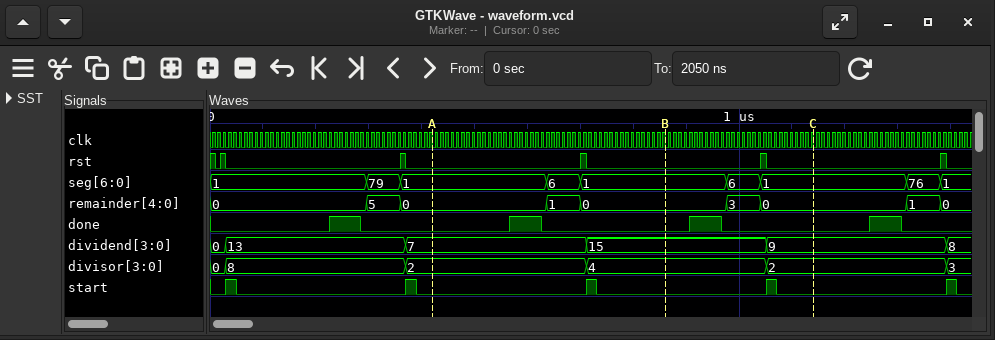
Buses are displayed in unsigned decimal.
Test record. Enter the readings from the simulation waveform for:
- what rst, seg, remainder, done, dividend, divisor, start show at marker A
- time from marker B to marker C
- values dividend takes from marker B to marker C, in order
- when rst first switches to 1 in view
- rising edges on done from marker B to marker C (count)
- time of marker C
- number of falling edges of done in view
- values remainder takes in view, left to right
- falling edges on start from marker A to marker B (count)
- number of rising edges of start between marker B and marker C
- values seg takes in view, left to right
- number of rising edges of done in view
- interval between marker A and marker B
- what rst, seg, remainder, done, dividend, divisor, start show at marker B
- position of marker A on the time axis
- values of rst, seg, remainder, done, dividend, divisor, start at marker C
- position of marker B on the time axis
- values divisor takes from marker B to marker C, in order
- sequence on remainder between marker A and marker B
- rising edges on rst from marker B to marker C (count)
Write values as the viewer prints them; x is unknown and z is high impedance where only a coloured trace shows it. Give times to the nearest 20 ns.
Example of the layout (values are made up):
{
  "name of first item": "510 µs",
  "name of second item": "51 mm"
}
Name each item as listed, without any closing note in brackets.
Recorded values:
{
  "what rst, seg, remainder, done, dividend, divisor, start show at marker A": "rst=0, seg=1, remainder=0, done=0, dividend=7, divisor=2, start=0",
  "time from marker B to marker C": "280 ns",
  "values dividend takes from marker B to marker C, in order": "15, 9",
  "when rst first switches to 1 in view": "20 ns",
  "rising edges on done from marker B to marker C": "1",
  "time of marker C": "1140 ns",
  "number of falling edges of done in view": "4",
  "values remainder takes in view, left to right": "0, 5, 0, 1, 0, 3, 0, 1, 0",
  "falling edges on start from marker A to marker B": "1",
  "number of rising edges of start between marker B and marker C": "1",
  "values seg takes in view, left to right": "1, 79, 1, 6, 1, 6, 1, 76, 1",
  "number of rising edges of done in view": "4",
  "interval between marker A and marker B": "440 ns",
  "what rst, seg, remainder, done, dividend, divisor, start show at marker B": "rst=0, seg=1, remainder=0, done=0, dividend=15, divisor=4, start=0",
  "position of marker A on the time axis": "420 ns",
  "values of rst, seg, remainder, done, dividend, divisor, start at marker C": "rst=0, seg=1, remainder=0, done=0, dividend=9, divisor=2, start=0",
  "position of marker B on the time axis": "860 ns",
  "values divisor takes from marker B to marker C, in order": "4, 2",
  "sequence on remainder between marker A and marker B": "0, 1, 0",
  "rising edges on rst from marker B to marker C": "1"
}
